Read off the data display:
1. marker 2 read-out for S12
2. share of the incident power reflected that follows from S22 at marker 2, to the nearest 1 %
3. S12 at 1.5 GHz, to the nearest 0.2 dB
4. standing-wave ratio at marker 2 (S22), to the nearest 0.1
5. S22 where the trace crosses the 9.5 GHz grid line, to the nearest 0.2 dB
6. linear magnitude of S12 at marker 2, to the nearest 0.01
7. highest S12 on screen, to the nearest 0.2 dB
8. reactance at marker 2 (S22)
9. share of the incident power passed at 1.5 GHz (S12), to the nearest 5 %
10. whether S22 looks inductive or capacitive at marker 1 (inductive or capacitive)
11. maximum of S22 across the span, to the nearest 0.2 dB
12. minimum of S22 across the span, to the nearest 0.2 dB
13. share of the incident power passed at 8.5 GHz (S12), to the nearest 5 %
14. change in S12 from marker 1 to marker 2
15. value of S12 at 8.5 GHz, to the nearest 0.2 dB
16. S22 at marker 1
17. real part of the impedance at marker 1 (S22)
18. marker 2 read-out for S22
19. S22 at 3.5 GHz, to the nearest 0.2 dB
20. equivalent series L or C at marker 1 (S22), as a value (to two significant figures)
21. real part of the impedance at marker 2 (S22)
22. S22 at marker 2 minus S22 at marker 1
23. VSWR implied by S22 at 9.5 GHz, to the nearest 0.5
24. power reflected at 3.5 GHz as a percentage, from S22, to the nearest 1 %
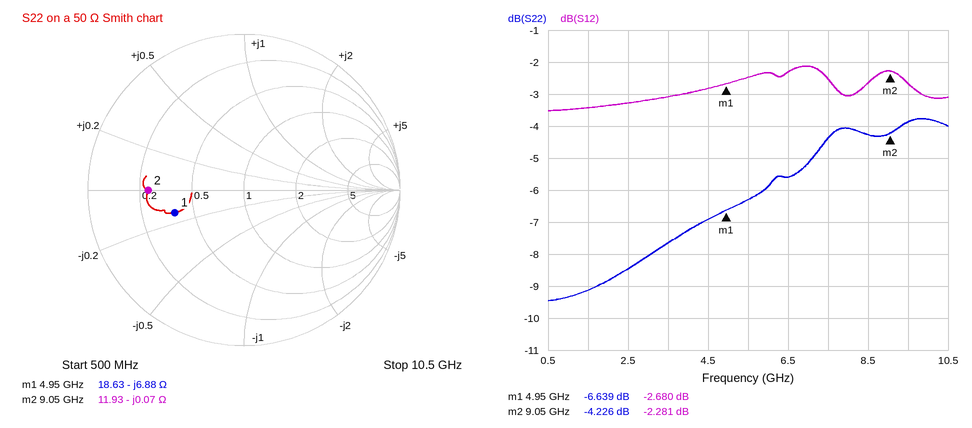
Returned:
-2.281 dB
38 %
-3.4 dB
4.2
-3.8 dB
0.77
-2.2 dB
-0.07 Ω
45 %
capacitive
-3.8 dB
-9.4 dB
55 %
0.399 dB
-2.6 dB
-6.639 dB
18.63 Ω
-4.226 dB
-7.6 dB
4.7 pF
11.93 Ω
2.413 dB
4.5
17 %
